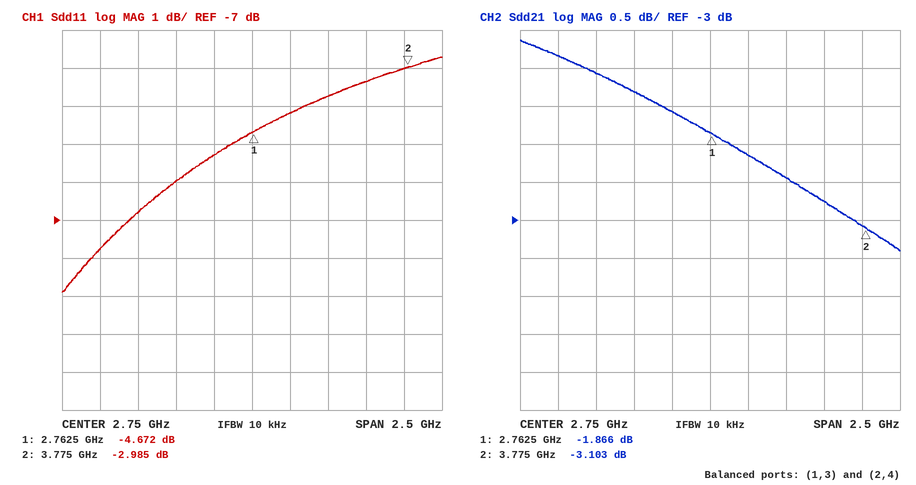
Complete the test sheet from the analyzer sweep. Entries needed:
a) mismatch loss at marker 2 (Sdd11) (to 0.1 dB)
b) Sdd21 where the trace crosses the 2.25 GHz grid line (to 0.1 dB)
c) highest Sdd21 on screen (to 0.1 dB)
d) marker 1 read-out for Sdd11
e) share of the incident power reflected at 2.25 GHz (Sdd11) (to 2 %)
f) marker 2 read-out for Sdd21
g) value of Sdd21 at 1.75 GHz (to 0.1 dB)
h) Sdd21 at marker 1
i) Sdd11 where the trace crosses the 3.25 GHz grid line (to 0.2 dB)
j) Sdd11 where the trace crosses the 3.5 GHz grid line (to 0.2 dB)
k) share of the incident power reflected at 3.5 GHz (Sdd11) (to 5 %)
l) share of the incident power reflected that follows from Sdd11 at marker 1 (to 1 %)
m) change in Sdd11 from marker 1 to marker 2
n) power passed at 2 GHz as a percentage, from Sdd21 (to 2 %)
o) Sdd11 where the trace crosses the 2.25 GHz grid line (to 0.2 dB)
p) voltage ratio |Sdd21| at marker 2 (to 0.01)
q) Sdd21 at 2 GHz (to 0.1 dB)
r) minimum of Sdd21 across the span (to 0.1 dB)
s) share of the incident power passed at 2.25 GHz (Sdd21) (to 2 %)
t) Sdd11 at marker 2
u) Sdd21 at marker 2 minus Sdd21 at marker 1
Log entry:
3.0 dB
-1.3 dB
-0.6 dB
-4.672 dB
26 %
-3.103 dB
-0.8 dB
-1.866 dB
-3.8 dB
-3.4 dB
45 %
34 %
1.687 dB
78 %
-6.0 dB
0.70
-1.1 dB
-3.4 dB
74 %
-2.985 dB
-1.237 dB
